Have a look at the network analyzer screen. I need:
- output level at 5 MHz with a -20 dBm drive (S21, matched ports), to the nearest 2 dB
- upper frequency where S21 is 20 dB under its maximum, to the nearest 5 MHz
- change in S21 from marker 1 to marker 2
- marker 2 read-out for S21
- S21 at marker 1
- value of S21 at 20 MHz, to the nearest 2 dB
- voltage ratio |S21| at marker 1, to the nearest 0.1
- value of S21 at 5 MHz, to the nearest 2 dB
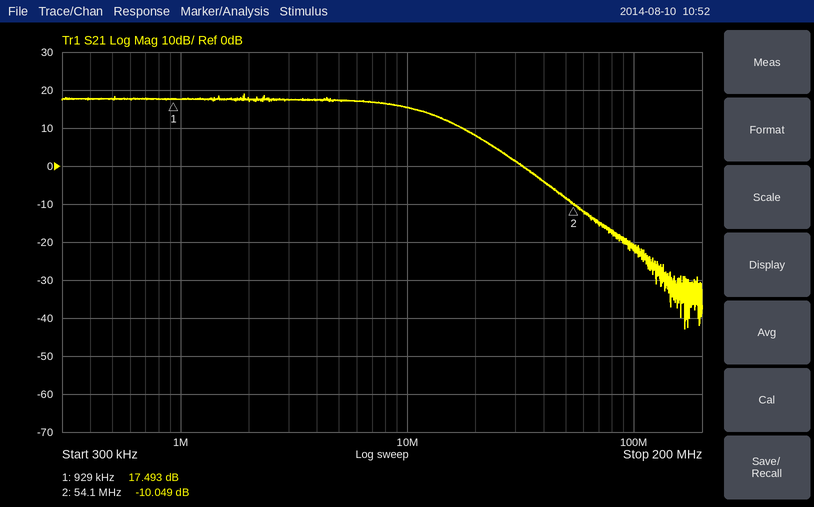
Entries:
-2 dBm
35 MHz
-27.542 dB
-10.049 dB
17.493 dB
8 dB
7.5
18 dB
